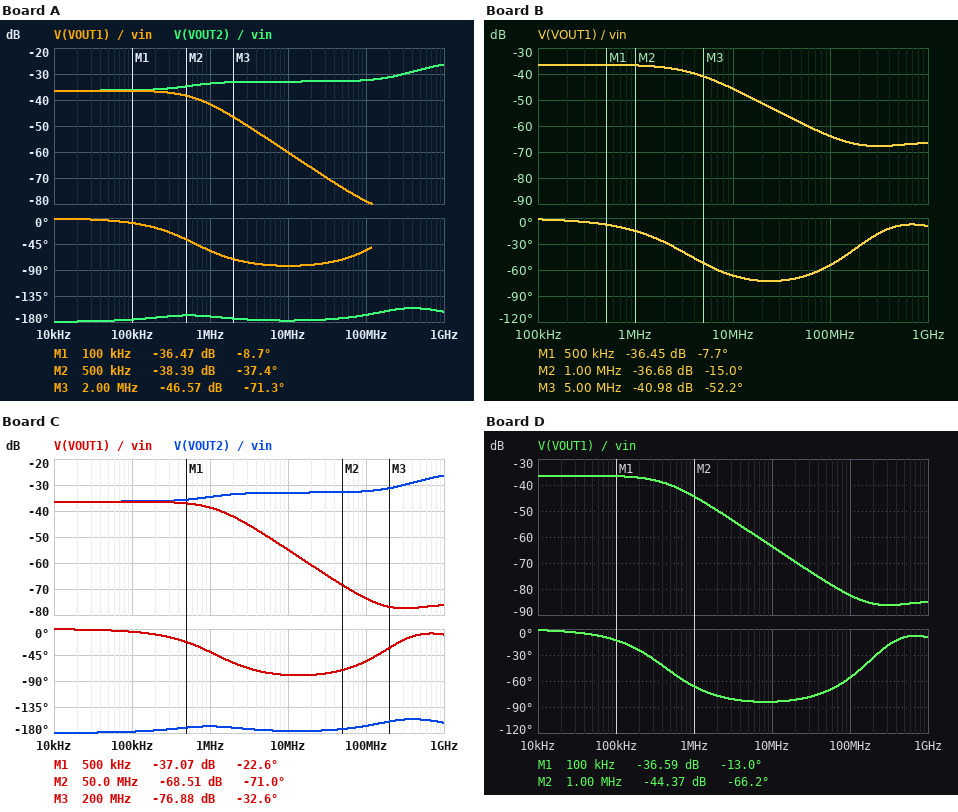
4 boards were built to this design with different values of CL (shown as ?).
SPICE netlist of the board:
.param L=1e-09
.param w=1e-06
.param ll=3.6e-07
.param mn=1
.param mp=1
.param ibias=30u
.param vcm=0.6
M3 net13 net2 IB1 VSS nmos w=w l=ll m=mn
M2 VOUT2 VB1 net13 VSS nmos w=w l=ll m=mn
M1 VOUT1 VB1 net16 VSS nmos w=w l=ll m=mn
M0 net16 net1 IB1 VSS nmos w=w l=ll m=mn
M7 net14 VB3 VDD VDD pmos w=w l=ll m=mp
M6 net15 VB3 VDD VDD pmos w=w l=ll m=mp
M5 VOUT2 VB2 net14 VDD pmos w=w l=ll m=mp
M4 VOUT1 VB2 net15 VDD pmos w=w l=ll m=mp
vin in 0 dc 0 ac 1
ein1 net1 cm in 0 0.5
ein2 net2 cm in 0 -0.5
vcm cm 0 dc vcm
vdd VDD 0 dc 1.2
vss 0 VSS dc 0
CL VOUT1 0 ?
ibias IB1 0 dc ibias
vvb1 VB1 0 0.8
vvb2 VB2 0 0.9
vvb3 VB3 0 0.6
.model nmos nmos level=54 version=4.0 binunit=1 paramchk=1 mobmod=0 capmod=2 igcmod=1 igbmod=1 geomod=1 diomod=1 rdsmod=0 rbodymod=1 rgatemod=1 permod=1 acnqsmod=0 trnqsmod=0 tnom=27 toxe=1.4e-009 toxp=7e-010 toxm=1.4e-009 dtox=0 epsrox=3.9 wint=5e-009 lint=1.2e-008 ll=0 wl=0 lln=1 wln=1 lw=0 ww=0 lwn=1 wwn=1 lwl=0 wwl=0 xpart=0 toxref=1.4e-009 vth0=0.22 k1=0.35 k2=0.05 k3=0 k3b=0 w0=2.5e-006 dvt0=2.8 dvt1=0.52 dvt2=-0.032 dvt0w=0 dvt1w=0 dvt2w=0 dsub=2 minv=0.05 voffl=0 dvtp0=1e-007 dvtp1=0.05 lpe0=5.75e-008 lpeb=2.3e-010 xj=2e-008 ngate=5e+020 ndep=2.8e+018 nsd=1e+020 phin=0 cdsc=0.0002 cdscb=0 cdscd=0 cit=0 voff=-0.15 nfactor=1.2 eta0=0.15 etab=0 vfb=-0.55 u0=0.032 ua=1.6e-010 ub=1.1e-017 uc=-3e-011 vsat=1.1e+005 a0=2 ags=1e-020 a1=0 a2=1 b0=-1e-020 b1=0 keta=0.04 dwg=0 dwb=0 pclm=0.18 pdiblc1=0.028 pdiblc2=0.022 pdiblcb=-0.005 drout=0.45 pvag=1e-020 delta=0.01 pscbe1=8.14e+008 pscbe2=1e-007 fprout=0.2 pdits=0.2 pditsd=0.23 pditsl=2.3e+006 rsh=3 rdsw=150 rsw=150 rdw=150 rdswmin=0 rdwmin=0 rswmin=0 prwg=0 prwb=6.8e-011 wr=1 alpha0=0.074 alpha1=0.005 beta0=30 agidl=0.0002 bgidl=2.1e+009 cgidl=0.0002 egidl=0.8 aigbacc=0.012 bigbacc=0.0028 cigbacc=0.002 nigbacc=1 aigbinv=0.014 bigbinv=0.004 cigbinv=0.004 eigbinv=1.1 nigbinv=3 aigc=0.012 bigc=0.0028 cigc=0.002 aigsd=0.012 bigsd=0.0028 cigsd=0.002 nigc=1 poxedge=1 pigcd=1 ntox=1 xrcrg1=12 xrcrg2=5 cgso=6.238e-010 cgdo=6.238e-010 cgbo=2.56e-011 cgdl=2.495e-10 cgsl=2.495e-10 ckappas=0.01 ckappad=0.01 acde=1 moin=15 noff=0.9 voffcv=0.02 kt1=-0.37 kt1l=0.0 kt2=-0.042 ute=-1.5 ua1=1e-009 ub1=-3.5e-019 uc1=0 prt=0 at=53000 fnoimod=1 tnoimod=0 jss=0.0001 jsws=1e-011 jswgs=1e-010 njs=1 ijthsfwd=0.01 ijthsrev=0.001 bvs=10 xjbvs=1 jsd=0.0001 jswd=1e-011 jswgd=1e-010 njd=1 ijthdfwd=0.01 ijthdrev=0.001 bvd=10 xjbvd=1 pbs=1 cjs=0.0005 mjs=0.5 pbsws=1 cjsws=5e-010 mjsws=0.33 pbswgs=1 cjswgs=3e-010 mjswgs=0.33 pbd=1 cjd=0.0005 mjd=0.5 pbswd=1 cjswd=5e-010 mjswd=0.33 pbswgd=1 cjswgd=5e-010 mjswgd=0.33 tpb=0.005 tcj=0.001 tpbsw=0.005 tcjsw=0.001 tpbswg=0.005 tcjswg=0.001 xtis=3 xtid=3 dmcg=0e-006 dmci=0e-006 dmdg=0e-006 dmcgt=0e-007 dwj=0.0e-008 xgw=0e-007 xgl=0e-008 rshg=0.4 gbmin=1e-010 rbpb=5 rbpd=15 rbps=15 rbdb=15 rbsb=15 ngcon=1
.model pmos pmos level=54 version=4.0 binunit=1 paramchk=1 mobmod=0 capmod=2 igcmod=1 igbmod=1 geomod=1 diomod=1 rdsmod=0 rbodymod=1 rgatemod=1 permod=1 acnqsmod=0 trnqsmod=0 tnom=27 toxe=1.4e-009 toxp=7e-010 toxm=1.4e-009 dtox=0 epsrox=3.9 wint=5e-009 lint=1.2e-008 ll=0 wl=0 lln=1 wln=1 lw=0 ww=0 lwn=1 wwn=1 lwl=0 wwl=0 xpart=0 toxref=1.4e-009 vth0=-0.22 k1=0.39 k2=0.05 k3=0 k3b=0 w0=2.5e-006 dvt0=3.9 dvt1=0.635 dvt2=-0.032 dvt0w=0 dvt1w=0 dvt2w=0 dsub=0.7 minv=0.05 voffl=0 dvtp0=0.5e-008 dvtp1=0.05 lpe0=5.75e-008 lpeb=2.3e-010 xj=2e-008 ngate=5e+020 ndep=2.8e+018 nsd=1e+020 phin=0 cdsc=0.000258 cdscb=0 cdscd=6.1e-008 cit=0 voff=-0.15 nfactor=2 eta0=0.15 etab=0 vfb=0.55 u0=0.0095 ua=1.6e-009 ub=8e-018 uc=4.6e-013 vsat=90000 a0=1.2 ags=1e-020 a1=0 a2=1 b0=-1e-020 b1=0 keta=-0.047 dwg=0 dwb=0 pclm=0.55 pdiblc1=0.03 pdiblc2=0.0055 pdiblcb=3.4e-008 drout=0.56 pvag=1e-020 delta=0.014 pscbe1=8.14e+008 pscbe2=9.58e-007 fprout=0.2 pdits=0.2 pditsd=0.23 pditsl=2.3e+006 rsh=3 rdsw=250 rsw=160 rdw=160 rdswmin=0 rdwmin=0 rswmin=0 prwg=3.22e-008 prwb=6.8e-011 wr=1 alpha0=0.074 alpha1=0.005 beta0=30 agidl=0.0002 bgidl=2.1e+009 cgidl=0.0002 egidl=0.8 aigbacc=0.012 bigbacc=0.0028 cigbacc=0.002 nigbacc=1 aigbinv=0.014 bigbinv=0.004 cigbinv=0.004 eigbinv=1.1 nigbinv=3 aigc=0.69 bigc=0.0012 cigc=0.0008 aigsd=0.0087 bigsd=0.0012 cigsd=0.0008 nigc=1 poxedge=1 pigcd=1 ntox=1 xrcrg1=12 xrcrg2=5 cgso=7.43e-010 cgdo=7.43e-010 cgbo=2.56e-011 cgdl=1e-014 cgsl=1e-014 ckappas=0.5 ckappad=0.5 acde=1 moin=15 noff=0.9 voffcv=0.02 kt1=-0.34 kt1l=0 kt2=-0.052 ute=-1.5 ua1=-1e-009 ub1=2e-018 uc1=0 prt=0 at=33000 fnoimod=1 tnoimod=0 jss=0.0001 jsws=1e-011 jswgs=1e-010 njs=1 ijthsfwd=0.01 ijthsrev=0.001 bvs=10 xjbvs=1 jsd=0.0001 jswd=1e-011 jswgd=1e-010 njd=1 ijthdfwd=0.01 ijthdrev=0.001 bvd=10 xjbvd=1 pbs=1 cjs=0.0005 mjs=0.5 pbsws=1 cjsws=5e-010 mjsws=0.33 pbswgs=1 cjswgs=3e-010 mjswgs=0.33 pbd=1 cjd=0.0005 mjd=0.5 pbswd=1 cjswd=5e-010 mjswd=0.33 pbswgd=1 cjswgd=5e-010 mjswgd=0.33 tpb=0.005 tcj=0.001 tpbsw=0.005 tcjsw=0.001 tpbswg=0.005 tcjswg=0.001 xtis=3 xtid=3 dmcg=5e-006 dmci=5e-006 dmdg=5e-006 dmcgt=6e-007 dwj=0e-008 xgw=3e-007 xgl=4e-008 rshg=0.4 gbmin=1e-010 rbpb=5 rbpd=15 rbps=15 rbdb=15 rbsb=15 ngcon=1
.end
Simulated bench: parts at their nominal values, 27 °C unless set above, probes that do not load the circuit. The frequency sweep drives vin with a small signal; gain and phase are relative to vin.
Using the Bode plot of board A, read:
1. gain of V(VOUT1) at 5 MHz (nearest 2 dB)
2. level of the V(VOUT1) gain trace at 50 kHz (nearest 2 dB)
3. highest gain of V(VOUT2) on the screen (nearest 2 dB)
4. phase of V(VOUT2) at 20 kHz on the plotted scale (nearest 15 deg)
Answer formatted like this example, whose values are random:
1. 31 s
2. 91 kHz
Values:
1. -54 dB
2. -36 dB
3. -26 dB
4. -180 deg
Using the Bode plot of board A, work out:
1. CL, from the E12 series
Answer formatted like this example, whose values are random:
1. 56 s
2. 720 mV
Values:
1. 22 pF
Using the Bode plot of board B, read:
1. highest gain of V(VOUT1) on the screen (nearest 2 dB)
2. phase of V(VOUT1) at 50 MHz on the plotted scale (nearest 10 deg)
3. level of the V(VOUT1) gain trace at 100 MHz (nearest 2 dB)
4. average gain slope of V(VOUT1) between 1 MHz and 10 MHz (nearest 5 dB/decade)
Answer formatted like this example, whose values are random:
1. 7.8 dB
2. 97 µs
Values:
1. -36 dB
2. -70 deg
3. -64 dB
4. -10 dB/decade
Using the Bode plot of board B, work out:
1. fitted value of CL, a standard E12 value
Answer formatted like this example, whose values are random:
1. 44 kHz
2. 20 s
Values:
1. 3.9 pF
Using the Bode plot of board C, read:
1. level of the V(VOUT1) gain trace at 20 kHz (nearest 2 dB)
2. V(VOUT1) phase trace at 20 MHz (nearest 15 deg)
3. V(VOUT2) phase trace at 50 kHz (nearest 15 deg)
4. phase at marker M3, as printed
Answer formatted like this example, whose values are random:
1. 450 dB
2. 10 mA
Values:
1. -36 dB
2. -75 deg
3. -180 deg
4. -32.6 deg
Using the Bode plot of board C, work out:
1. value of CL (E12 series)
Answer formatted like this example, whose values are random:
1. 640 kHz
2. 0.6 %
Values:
1. 12 pF
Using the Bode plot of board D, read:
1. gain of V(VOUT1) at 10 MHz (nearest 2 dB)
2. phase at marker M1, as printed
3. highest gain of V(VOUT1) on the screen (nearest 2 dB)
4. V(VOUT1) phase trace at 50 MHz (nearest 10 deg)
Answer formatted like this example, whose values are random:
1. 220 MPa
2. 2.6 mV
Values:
1. -64 dB
2. -13.0 deg
3. -36 dB
4. -70 deg
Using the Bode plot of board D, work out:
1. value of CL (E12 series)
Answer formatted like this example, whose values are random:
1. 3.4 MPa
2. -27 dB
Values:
1. 33 pF
